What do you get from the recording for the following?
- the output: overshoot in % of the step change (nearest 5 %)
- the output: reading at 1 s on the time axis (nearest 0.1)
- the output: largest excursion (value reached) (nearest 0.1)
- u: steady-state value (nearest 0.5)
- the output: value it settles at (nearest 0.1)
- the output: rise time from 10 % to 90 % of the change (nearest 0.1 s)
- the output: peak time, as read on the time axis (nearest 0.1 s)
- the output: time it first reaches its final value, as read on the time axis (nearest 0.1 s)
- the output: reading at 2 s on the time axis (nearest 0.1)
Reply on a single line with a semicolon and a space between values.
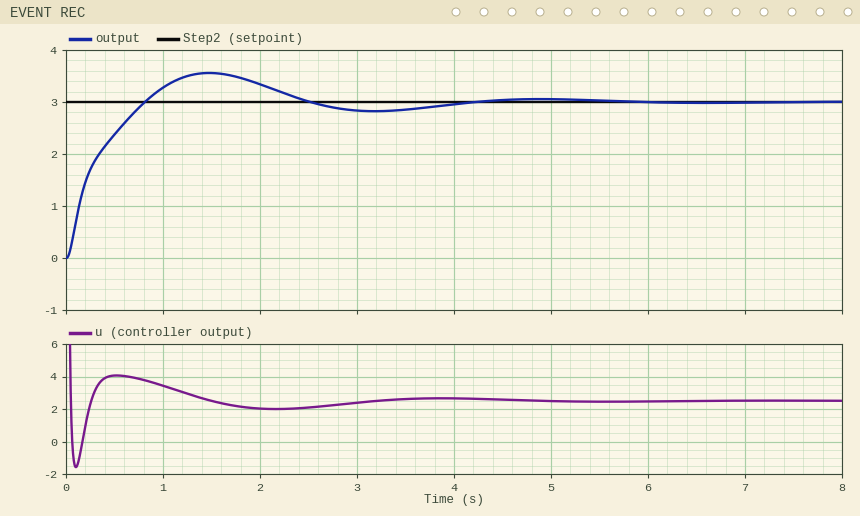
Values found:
20 %; 3.3; 3.6; 2.5; 3.0; 0.6 s; 1.5 s; 0.8 s; 3.3
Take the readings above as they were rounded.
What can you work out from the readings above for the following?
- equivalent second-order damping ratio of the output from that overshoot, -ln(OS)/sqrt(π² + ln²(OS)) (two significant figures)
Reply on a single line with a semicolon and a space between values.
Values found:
0.46
